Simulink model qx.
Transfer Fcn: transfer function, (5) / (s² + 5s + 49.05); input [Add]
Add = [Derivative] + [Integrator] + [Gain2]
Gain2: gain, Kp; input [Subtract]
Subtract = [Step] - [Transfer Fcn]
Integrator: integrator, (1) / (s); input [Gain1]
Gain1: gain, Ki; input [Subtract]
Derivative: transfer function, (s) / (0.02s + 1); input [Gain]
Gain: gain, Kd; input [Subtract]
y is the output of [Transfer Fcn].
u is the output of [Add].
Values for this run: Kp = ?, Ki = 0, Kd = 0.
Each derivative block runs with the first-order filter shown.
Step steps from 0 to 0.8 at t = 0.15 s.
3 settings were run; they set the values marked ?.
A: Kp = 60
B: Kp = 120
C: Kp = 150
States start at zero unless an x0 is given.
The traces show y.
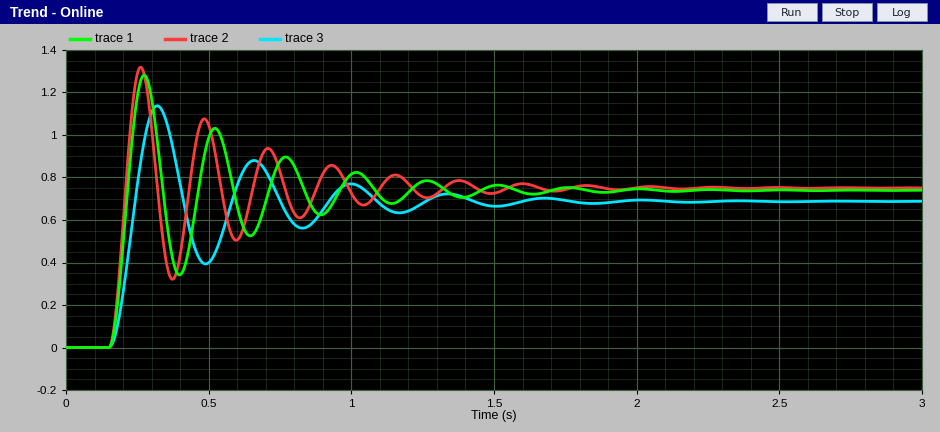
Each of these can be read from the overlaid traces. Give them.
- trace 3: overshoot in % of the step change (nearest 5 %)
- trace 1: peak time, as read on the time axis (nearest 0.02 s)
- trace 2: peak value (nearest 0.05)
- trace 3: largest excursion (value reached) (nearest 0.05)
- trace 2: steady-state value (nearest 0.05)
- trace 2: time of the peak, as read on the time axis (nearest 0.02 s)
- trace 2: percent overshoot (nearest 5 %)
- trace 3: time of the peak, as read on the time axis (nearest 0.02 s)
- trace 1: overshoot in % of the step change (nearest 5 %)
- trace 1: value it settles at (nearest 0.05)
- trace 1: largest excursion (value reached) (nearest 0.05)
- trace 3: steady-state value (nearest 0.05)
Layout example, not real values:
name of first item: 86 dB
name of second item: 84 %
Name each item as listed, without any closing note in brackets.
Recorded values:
trace 3: overshoot in % of the step change: 65 %
trace 1: peak time, as read on the time axis: 0.28 s
trace 2: peak value: 1.30
trace 3: largest excursion (value reached): 1.15
trace 2: steady-state value: 0.75
trace 2: time of the peak, as read on the time axis: 0.26 s
trace 2: percent overshoot: 75 %
trace 3: time of the peak, as read on the time axis: 0.32 s
trace 1: overshoot in % of the step change: 75 %
trace 1: value it settles at: 0.75
trace 1: largest excursion (value reached): 1.30
trace 3: steady-state value: 0.70
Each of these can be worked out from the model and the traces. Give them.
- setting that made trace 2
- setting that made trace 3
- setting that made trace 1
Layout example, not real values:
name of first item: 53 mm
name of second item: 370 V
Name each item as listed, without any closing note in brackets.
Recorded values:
setting that made trace 2: C
setting that made trace 3: A
setting that made trace 1: B
